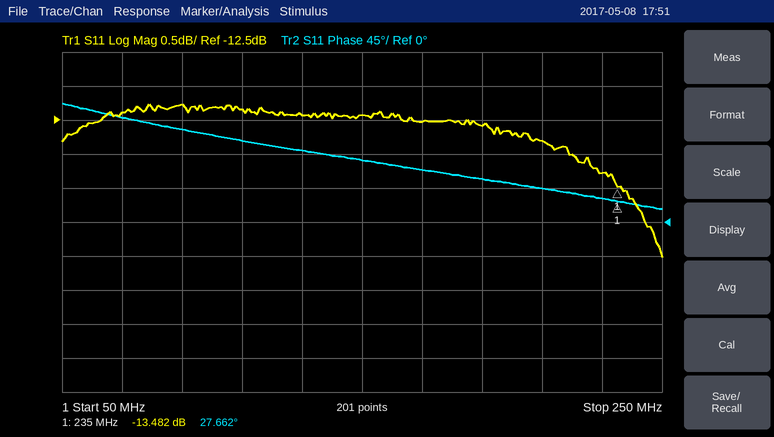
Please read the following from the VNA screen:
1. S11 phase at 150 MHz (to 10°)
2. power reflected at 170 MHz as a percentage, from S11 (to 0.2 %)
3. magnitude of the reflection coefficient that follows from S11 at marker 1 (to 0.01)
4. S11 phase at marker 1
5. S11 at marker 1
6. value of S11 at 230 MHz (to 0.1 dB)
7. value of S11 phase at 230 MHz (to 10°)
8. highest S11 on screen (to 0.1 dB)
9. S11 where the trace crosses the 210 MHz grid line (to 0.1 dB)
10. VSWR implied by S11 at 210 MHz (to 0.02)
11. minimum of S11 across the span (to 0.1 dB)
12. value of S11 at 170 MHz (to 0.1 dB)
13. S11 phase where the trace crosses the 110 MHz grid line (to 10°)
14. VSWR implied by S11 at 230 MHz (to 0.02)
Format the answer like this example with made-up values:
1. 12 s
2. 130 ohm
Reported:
1. 80°
2. 5.6 %
3. 0.21
4. 27.662°
5. -13.482 dB
6. -13.3 dB
7. 30°
8. -12.3 dB
9. -12.8 dB
10. 1.60
11. -14.5 dB
12. -12.5 dB
13. 110°
14. 1.56
